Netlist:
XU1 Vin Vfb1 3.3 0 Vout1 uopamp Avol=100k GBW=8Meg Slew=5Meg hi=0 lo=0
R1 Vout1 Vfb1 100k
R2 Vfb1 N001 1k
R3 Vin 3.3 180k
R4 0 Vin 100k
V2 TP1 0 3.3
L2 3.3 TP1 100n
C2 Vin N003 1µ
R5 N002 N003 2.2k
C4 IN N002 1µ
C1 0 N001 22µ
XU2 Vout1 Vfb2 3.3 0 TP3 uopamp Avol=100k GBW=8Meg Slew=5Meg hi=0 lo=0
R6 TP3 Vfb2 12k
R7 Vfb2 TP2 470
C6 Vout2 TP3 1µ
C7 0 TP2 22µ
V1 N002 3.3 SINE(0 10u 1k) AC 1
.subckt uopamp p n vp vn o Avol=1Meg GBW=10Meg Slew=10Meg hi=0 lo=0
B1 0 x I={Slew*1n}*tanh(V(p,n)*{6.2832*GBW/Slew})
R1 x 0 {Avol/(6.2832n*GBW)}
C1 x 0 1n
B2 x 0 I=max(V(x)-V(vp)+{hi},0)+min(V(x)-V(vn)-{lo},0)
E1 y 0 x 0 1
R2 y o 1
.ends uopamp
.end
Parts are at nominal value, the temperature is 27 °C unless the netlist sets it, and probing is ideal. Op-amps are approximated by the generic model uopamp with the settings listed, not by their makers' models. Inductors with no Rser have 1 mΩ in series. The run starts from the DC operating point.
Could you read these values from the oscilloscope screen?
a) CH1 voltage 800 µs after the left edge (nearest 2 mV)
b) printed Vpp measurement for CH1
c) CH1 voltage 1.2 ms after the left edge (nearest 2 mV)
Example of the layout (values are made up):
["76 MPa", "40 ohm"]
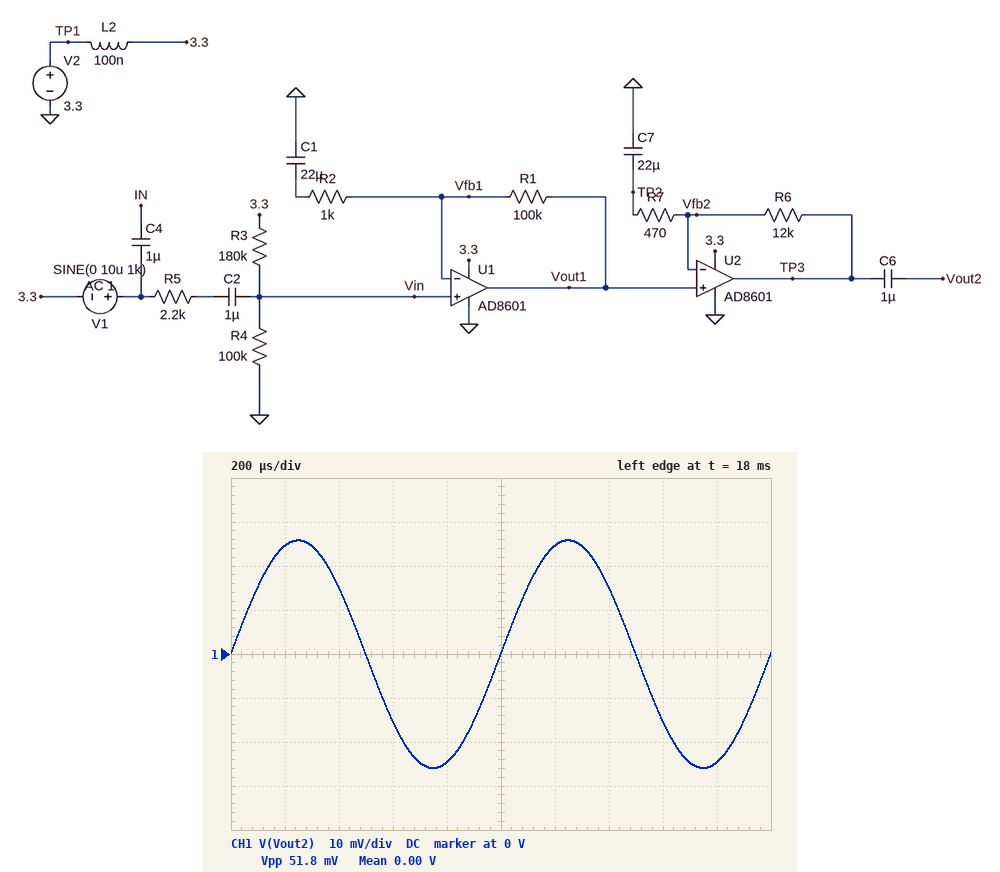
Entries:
["-24 mV", "51.8 mV", "24 mV"]
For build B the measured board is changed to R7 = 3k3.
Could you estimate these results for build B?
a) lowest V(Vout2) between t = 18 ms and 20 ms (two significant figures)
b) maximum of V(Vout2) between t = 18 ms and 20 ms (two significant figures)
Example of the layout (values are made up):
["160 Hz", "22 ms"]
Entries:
["-4.5 mV", "4.5 mV"]
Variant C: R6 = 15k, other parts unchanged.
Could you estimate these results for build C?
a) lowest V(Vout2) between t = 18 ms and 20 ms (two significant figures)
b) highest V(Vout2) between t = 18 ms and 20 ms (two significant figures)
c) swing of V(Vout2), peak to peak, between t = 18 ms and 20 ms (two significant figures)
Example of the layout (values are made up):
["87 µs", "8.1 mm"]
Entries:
["-32 mV", "32 mV", "64 mV"]
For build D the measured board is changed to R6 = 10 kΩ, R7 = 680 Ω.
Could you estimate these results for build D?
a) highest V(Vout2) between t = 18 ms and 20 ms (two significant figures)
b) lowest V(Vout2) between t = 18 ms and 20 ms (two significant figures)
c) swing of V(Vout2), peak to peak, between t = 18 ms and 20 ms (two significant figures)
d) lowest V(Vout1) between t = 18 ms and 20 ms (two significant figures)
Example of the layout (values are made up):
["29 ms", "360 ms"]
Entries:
["15 mV", "-15 mV", "31 mV", "1.2 V"]
